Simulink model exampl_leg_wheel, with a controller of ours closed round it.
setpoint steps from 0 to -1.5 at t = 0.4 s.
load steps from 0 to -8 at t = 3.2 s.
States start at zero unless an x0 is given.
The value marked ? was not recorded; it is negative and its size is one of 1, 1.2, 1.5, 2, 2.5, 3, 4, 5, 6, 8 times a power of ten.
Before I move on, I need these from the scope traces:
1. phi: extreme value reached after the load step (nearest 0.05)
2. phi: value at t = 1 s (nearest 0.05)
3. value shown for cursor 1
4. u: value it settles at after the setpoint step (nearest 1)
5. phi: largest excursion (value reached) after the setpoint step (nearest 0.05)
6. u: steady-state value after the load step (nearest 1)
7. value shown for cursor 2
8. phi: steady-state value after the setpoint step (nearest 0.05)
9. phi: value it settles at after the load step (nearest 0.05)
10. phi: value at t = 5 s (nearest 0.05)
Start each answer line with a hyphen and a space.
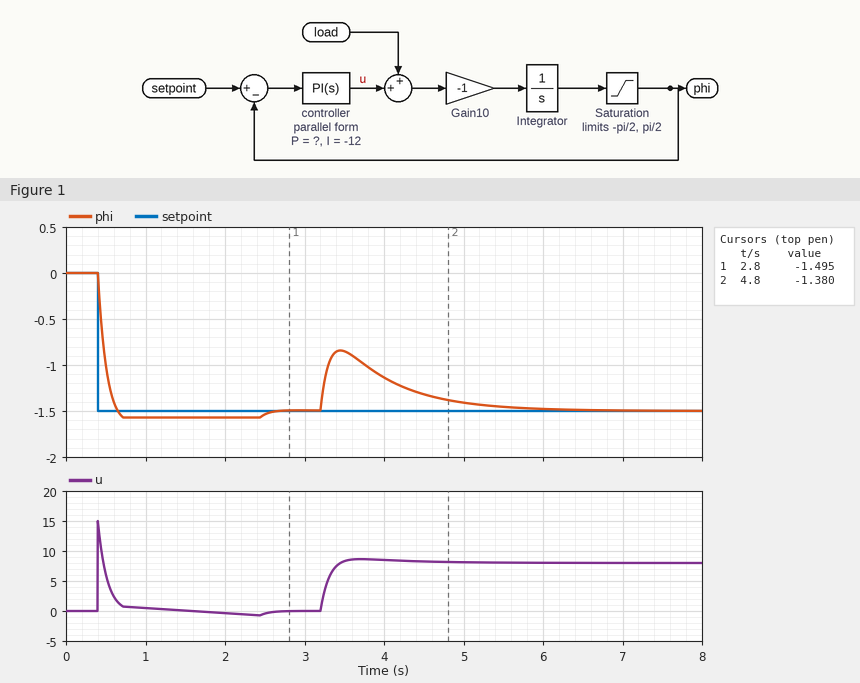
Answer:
- -0.85
- -1.55
- -1.495
- 0
- -1.55
- 8
- -1.380
- -1.50
- -1.50
- -1.40
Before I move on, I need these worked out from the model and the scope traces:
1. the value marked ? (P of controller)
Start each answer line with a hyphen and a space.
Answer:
- -10
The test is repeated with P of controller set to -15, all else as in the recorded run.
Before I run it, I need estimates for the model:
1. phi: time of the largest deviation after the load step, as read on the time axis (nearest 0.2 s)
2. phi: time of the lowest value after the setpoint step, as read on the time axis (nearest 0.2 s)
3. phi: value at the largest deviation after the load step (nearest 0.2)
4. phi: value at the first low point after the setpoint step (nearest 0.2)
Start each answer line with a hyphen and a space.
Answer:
- 3.4 s
- 0.8 s
- -1.0
- -1.6
